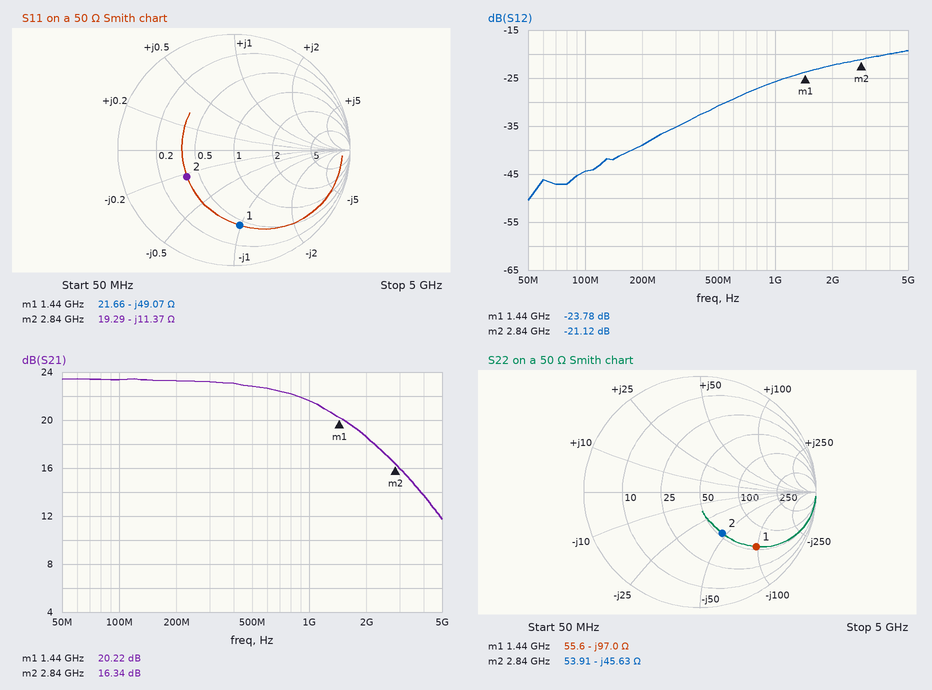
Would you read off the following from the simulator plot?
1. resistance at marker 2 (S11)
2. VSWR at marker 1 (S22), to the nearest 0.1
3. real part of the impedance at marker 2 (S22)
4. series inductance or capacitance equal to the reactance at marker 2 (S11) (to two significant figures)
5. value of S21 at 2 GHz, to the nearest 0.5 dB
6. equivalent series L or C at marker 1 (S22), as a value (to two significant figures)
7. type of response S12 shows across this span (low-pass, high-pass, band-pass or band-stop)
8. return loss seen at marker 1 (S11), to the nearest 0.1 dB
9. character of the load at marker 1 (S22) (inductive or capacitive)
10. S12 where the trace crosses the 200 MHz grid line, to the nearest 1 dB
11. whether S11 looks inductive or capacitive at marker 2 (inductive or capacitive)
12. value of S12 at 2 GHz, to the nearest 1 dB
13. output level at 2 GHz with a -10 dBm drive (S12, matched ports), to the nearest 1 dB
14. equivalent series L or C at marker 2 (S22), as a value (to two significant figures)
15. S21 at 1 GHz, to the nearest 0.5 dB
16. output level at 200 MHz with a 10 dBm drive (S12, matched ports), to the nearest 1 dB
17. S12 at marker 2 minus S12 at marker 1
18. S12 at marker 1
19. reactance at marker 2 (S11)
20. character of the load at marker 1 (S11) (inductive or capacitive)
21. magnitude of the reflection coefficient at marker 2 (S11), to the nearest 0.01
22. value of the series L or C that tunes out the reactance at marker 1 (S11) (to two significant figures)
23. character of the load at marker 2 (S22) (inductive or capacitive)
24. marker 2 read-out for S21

19.29 Ω
5.2
53.91 Ω
4.9 pF
18.5 dB
1.1 pF
high-pass
3.7 dB
capacitive
-39 dB
capacitive
-22 dB
-32 dBm
1.2 pF
21.5 dB
-29 dBm
2.66 dB
-23.78 dB
-11.37 Ω
capacitive
0.47
5.4 nH
capacitive
16.34 dB
